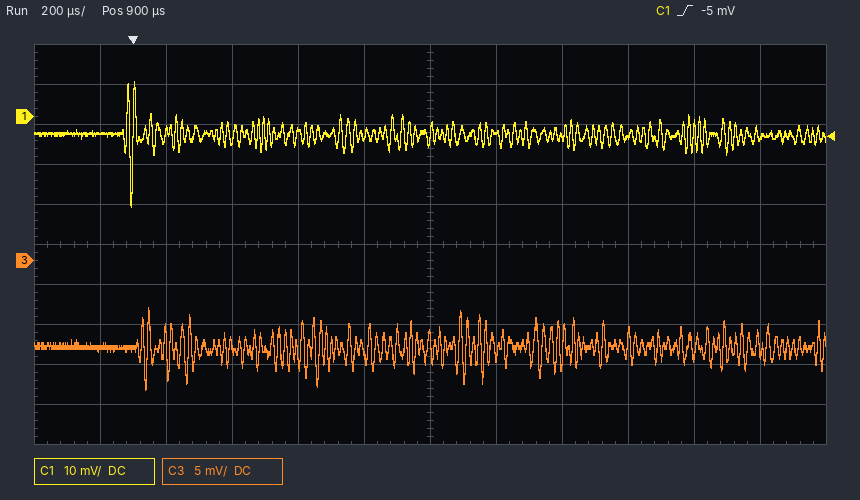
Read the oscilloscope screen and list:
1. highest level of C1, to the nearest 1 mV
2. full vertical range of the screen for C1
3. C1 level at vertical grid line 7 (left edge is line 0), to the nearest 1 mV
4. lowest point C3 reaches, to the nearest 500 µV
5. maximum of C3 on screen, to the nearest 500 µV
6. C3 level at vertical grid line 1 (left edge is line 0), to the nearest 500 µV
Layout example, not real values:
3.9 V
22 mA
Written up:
9 mV
100 mV
-4 mV
-16.0 mV
-6.0 mV
-11.0 mV
